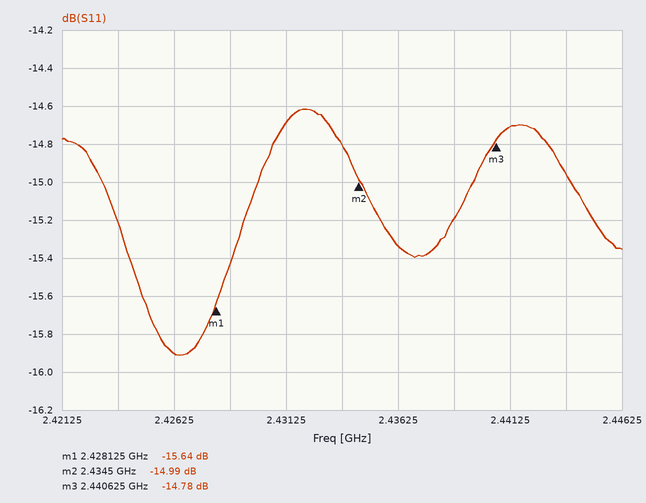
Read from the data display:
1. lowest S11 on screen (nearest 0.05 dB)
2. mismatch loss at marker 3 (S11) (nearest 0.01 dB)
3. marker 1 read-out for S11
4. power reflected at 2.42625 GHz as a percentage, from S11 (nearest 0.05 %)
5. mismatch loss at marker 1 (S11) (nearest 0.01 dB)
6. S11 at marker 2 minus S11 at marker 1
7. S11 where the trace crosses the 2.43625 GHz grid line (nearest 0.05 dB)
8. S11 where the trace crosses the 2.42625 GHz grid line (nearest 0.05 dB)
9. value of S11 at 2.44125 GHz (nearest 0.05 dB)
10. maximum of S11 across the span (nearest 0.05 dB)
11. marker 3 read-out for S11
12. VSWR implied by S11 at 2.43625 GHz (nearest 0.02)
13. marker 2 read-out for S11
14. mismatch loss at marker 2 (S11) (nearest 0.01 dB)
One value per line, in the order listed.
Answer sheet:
-15.90 dB
0.15 dB
-15.64 dB
2.55 %
0.12 dB
0.65 dB
-15.35 dB
-15.90 dB
-14.70 dB
-14.60 dB
-14.78 dB
1.42
-14.99 dB
0.14 dB
